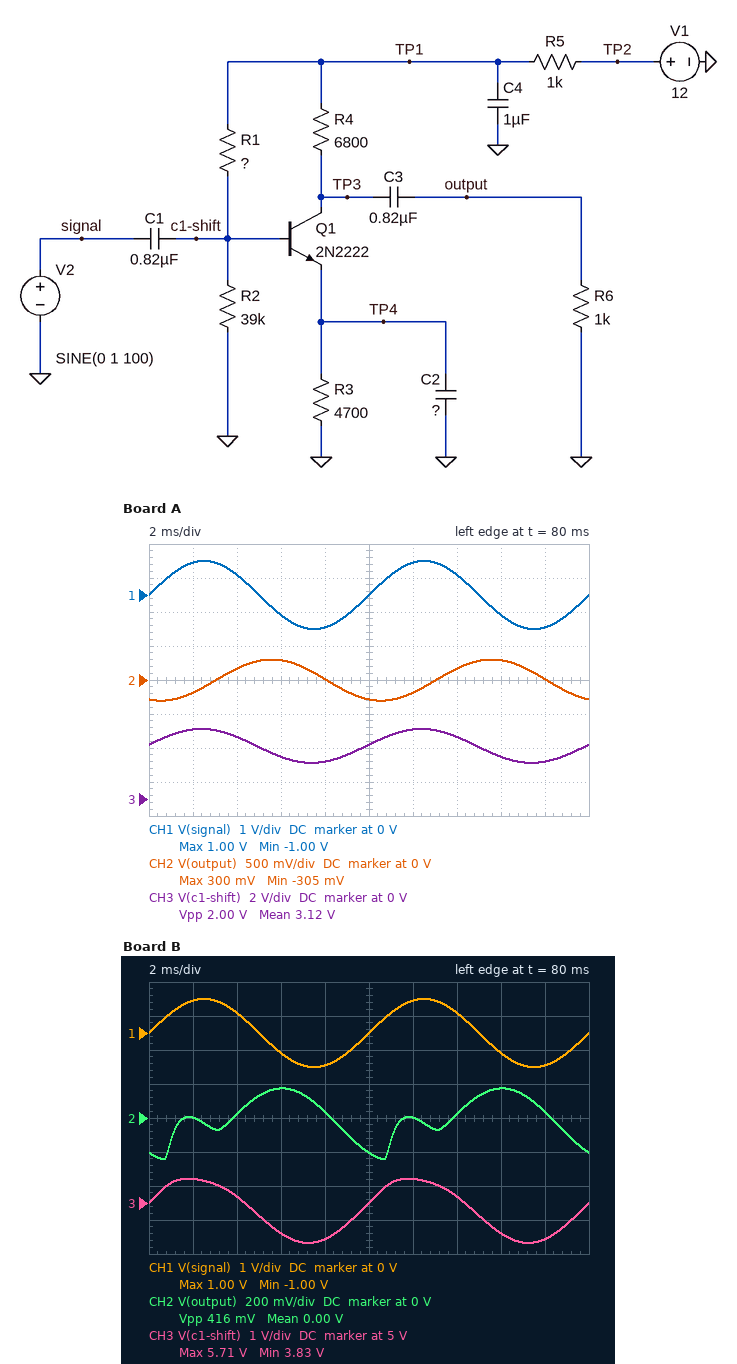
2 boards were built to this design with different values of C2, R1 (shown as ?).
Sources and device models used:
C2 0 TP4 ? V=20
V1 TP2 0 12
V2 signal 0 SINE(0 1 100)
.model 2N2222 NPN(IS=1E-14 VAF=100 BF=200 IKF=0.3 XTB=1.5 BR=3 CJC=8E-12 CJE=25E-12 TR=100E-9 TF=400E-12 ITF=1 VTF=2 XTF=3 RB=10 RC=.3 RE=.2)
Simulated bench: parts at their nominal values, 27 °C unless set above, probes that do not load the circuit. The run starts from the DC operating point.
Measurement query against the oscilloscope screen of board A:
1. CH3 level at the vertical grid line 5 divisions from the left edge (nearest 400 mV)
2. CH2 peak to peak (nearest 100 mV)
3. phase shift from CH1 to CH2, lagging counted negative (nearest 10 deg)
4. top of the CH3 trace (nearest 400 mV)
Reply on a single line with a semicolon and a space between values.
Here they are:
3.2 V; 600 mV; -110 deg; 4.0 V
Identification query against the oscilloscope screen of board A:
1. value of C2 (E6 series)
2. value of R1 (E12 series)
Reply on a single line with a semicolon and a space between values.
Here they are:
470 nF; 100 kΩ
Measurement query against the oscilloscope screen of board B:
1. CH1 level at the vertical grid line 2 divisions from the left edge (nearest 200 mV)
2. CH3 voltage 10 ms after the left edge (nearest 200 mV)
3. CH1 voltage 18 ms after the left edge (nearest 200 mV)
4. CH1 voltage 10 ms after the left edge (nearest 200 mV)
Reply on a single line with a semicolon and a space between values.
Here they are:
600 mV; 5.0 V; -1.0 V; 0 V
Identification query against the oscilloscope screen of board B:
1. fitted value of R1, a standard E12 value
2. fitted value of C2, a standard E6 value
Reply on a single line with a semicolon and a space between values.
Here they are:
39 kΩ; 220 nF
